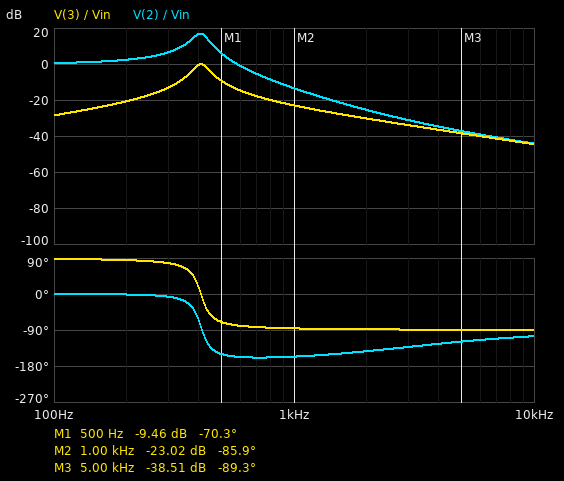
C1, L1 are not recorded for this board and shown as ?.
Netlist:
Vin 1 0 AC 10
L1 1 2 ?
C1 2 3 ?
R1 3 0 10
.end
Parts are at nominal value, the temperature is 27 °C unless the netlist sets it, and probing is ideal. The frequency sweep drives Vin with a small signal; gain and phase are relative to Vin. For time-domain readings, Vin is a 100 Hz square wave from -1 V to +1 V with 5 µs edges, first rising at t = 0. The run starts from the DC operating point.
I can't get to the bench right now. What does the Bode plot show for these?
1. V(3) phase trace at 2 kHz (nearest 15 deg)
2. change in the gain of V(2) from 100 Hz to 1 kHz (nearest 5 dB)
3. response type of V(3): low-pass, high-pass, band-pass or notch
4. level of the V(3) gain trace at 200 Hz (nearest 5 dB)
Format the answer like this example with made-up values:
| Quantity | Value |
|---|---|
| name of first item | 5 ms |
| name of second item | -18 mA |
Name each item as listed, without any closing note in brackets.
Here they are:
| Quantity | Value |
|---|---|
| V(3) phase trace at 2 kHz | -90 deg |
| change in the gain of V(2) from 100 Hz to 1 kHz | -15 dB |
| response type of V(3): low-pass, high-pass, band-pass or notch | band-pass |
| level of the V(3) gain trace at 200 Hz | -20 dB |
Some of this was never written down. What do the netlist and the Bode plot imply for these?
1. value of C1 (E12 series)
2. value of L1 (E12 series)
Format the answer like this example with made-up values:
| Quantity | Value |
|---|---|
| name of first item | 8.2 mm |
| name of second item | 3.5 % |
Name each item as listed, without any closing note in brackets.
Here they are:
| Quantity | Value |
|---|---|
| value of C1 | 5.6 µF |
| value of L1 | 27 mH |
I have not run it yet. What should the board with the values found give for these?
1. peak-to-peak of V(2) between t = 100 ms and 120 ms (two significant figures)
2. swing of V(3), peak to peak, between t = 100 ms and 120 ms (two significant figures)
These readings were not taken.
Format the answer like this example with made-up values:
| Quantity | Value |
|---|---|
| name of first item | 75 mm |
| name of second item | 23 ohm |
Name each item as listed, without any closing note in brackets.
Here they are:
| Quantity | Value |
|---|---|
| peak-to-peak of V(2) between t = 100 ms and 120 ms | 4.3 V |
| swing of V(3), peak to peak, between t = 100 ms and 120 ms | 370 mV |
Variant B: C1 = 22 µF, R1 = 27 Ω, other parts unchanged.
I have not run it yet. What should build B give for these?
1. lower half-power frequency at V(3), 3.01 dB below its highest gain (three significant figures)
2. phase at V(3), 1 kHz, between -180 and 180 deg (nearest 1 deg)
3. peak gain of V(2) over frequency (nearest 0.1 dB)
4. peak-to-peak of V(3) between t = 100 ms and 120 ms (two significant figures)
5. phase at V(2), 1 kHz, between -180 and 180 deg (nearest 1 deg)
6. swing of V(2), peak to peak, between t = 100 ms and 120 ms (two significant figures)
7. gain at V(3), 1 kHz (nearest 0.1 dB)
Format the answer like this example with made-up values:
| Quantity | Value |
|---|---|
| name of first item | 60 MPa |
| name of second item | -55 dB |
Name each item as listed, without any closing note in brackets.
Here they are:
| Quantity | Value |
|---|---|
| lower half-power frequency at V(3), 3.01 dB below its highest gain | 142 Hz |
| phase at V(3), 1 kHz, between -180 and 180 deg | -81 deg |
| peak gain of V(2) over frequency | 4.6 dB |
| peak-to-peak of V(3) between t = 100 ms and 120 ms | 1.8 V |
| phase at V(2), 1 kHz, between -180 and 180 deg | -96 deg |
| swing of V(2), peak to peak, between t = 100 ms and 120 ms | 3.4 V |
| gain at V(3), 1 kHz | -15.7 dB |
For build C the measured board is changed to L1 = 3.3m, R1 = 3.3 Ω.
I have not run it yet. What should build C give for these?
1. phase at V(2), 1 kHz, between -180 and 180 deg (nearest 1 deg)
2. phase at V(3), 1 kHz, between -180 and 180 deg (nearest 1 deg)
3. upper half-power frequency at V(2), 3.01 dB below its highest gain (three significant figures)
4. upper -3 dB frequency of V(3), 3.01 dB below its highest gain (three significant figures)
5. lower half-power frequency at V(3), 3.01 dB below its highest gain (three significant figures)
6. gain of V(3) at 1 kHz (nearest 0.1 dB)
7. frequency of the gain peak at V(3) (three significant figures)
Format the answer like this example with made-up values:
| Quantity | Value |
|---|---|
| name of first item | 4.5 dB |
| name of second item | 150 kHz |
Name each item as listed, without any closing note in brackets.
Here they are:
| Quantity | Value |
|---|---|
| phase at V(2), 1 kHz, between -180 and 180 deg | -17 deg |
| phase at V(3), 1 kHz, between -180 and 180 deg | 67 deg |
| upper half-power frequency at V(2), 3.01 dB below its highest gain | 1.24 kHz |
| upper -3 dB frequency of V(3), 3.01 dB below its highest gain | 1.25 kHz |
| lower half-power frequency at V(3), 3.01 dB below its highest gain | 1.09 kHz |
| gain of V(3) at 1 kHz | -8.1 dB |
| frequency of the gain peak at V(3) | 1.17 kHz |
